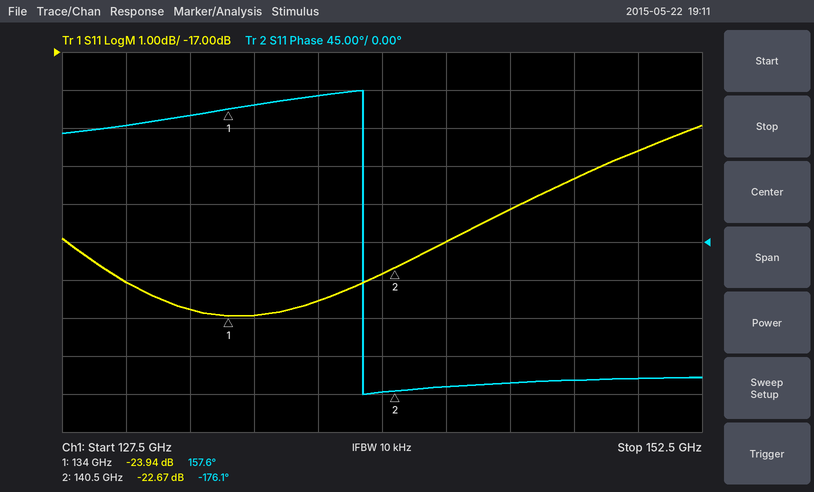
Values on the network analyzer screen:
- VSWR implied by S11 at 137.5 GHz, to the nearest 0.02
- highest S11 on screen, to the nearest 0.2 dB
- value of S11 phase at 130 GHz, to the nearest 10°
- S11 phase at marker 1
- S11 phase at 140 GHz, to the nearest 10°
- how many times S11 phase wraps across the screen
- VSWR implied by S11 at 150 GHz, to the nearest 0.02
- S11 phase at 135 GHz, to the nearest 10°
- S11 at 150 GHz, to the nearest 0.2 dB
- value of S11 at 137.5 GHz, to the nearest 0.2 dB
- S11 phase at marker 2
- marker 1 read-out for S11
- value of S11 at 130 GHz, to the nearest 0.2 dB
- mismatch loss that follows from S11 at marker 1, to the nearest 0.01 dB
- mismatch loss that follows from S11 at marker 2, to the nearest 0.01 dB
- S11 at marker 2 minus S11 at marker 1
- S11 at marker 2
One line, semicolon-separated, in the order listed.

1.14; -19.0 dB; 140°; 157.6°; -180°; 1; 1.24; 160°; -19.6 dB; -23.6 dB; -176.1°; -23.94 dB; -23.0 dB; 0.02 dB; 0.02 dB; 1.27 dB; -22.67 dB
